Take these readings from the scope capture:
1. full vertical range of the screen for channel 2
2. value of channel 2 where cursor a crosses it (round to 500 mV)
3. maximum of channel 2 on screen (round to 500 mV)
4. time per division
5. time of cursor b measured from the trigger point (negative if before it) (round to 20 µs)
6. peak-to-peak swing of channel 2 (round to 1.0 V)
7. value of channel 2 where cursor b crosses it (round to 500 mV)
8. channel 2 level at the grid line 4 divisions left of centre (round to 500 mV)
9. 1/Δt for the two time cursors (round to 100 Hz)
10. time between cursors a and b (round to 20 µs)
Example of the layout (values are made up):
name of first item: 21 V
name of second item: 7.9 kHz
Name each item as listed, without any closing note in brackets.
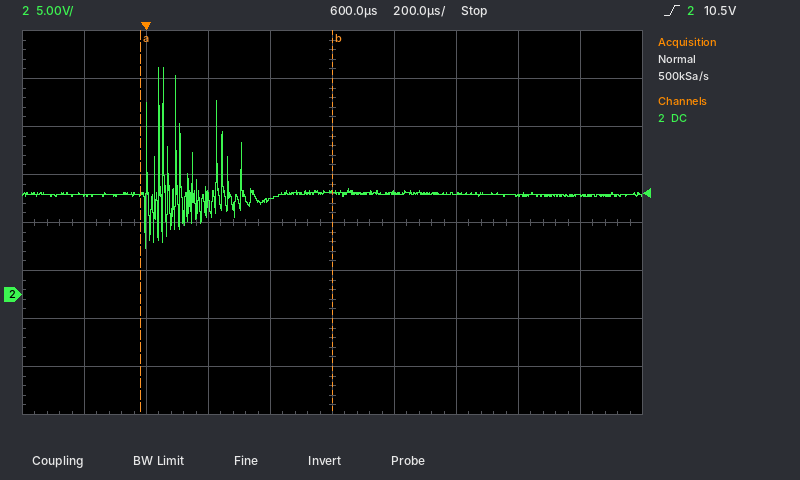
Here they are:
full vertical range of the screen for channel 2: 40 V
value of channel 2 where cursor a crosses it: 10.5 V
maximum of channel 2 on screen: 23.5 V
time per division: 200 µs
time of cursor b measured from the trigger point (negative if before it): +600 µs
peak-to-peak swing of channel 2: 19.0 V
value of channel 2 where cursor b crosses it: 10.5 V
channel 2 level at the grid line 4 divisions left of centre: 10.5 V
1/Δt for the two time cursors: 1.6 kHz
time between cursors a and b: 620 µs
